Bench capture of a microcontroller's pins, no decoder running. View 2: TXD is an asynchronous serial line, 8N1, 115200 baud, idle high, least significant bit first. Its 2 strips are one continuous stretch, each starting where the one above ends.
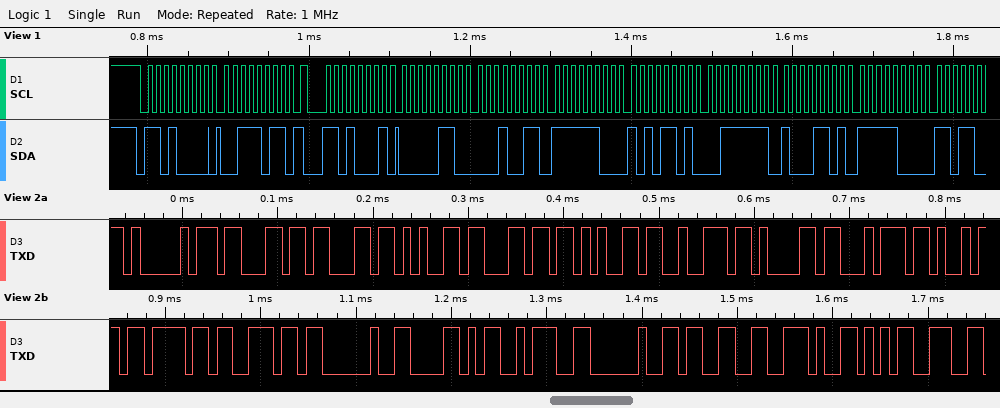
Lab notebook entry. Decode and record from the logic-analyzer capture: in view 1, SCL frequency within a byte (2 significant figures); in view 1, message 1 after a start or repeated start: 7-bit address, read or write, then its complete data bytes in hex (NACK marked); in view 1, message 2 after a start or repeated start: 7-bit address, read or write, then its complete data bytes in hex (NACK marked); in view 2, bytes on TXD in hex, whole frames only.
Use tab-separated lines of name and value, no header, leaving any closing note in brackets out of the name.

in view 1, SCL frequency within a byte	100 kHz
in view 1, message 1 after a start or repeated start: 7-bit address, read or write, then its complete data bytes in hex	0x68 write: 3B
in view 1, message 2 after a start or repeated start: 7-bit address, read or write, then its complete data bytes in hex	0x68 read: 06 13 FC AD 3F 8D F8
in view 2, bytes on TXD in hex, whole frames only	41 63 63 65 6C 65 72 61 74 69 6F 6E 20 58 3A 20 33 2E 35
